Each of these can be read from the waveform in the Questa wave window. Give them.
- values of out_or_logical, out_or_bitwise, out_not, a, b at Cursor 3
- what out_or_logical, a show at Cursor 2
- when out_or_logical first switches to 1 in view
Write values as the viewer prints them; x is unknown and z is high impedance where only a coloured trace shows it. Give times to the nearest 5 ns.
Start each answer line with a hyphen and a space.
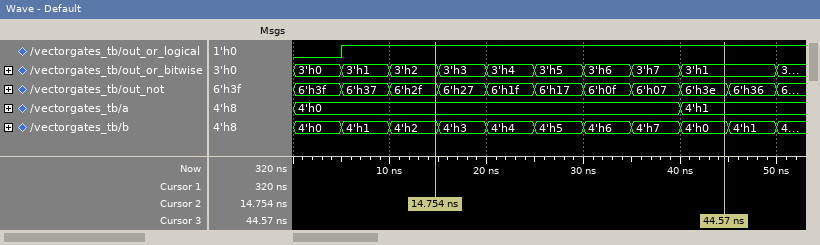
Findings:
- out_or_logical=1, out_or_bitwise=3'h1, out_not=6'h3e, a=4'h1, b=4'h0
- out_or_logical=1, a=4'h0
- 5 ns
